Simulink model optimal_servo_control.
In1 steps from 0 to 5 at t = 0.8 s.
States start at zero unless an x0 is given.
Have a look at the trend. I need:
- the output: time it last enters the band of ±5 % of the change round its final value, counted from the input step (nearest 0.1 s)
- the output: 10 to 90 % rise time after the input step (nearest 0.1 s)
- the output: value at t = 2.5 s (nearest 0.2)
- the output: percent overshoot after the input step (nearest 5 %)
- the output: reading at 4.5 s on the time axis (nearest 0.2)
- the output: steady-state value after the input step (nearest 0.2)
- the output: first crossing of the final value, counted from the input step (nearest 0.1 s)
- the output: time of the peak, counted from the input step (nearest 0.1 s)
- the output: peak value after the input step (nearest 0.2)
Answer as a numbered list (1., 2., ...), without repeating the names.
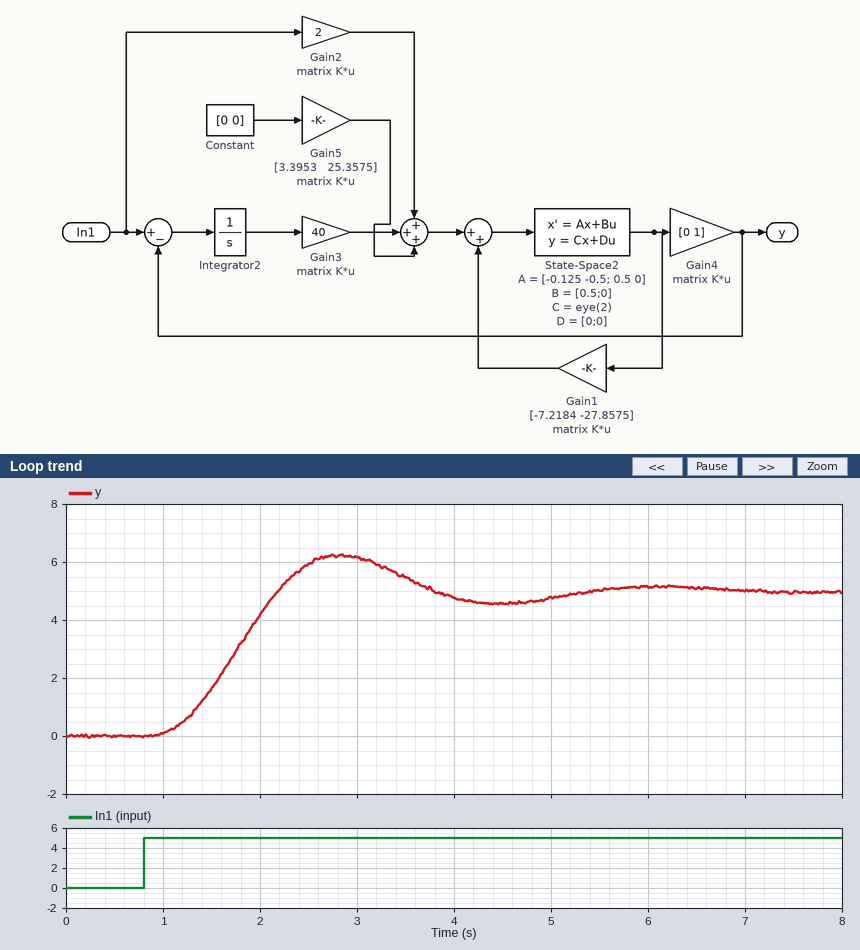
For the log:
1. 4.2 s
2. 0.9 s
3. 6.0
4. 25 %
5. 4.6
6. 5.0
7. 1.4 s
8. 2.0 s
9. 6.2
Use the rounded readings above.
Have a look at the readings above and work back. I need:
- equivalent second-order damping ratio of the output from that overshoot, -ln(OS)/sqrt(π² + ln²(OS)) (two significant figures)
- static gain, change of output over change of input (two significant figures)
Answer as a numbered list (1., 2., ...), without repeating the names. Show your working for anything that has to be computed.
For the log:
1. ln(0.25) = -1.386; 1.386 / sqrt(9.870 + 1.922) = 0.40
2. (5 - 0) / (5 - 0) = 1.0
